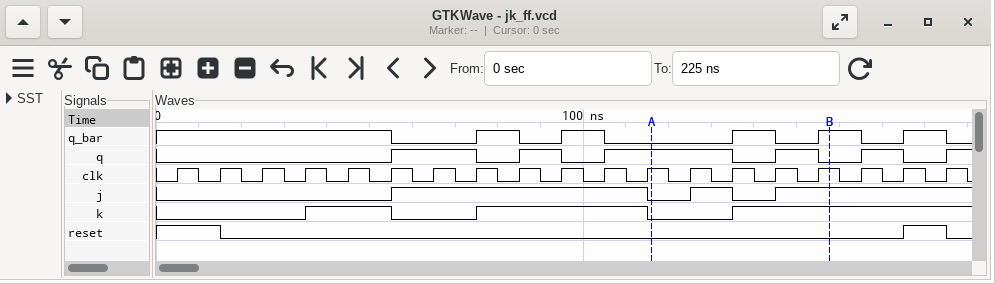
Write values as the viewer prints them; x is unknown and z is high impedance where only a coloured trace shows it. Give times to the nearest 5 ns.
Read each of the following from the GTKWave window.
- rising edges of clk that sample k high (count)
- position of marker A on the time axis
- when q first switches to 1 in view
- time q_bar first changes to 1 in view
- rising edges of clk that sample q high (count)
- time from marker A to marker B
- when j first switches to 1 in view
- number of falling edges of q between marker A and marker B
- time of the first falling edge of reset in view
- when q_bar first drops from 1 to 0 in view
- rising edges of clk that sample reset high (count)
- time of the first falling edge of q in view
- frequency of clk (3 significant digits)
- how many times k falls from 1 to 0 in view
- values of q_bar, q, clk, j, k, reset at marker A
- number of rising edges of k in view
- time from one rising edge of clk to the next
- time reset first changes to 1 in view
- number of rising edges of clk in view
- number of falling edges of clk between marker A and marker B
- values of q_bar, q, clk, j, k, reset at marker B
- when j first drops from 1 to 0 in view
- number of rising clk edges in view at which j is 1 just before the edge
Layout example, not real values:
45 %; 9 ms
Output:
11; 115 ns; 55 ns; 75 ns; 8; 40 ns; 55 ns; 2; 15 ns; 55 ns; 3; 75 ns; 100 MHz; 2; q_bar=0, q=1, clk=1, j=0, k=0, reset=0; 3; 10 ns; 175 ns; 19; 4; q_bar=1, q=0, clk=1, j=1, k=1, reset=0; 115 ns; 11
